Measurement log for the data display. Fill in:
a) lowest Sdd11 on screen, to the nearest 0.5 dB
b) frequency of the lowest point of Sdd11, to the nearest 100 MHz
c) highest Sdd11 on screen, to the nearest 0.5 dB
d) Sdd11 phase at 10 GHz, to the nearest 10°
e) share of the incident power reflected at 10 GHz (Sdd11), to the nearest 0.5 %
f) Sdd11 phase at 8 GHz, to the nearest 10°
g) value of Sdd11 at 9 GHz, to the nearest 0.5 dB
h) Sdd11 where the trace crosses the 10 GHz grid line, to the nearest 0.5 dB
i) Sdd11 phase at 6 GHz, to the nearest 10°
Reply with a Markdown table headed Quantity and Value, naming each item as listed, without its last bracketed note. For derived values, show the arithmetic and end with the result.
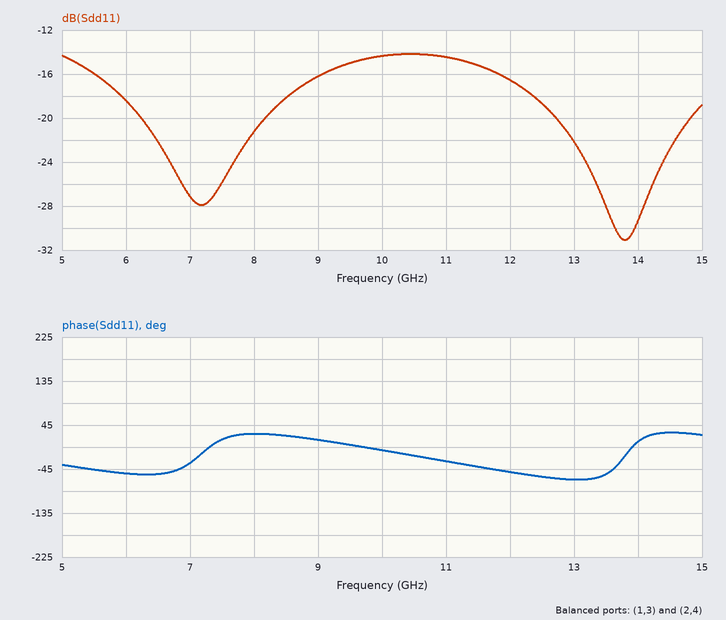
| Quantity | Value |
|---|---|
| lowest Sdd11 on screen, to the nearest 0.5 dB | -31.0 dB |
| frequency of the lowest point of Sdd11, to the nearest 100 MHz | 13.8 GHz |
| highest Sdd11 on screen, to the nearest 0.5 dB | -14.0 dB |
| Sdd11 phase at 10 GHz, to the nearest 10° | -10° |
| share of the incident power reflected at 10 GHz (Sdd11), to the nearest 0.5 % | 10^(-14.5/10) ≈ 3.5 % |
| Sdd11 phase at 8 GHz, to the nearest 10° | 30° |
| value of Sdd11 at 9 GHz, to the nearest 0.5 dB | -16.0 dB |
| Sdd11 where the trace crosses the 10 GHz grid line, to the nearest 0.5 dB | -14.5 dB |
| Sdd11 phase at 6 GHz, to the nearest 10° | -50° |
